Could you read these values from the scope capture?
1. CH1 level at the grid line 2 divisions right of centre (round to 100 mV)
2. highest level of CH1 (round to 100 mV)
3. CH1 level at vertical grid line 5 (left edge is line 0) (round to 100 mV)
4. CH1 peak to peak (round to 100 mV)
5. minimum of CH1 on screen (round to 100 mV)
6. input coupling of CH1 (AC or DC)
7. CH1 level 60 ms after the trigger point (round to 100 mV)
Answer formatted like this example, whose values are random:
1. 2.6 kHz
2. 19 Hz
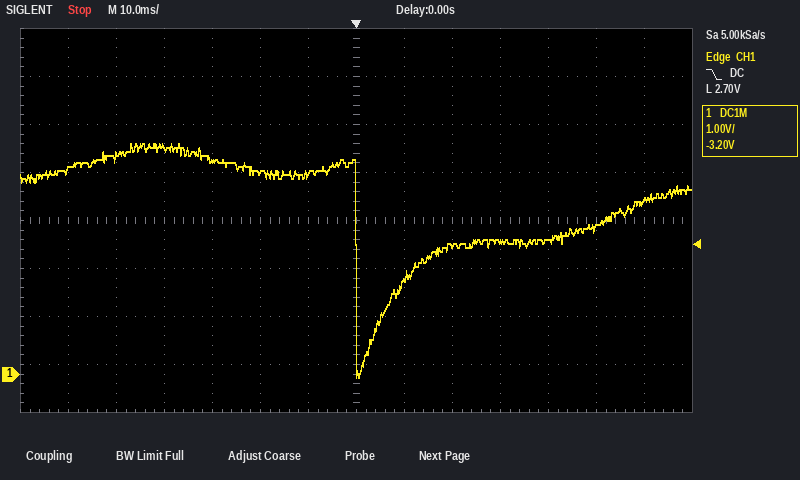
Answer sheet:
1. 2.7 V
2. 4.8 V
3. 4.2 V
4. 4.9 V
5. -100 mV
6. DC
7. 3.6 V
